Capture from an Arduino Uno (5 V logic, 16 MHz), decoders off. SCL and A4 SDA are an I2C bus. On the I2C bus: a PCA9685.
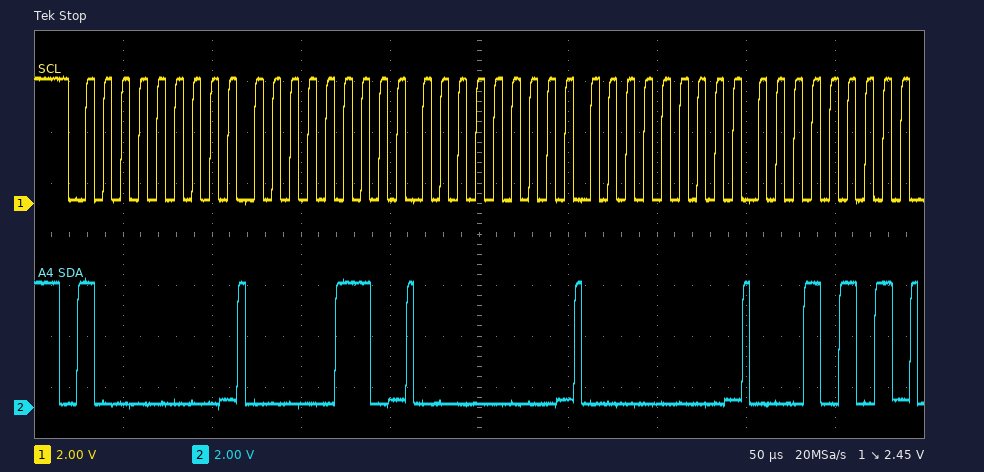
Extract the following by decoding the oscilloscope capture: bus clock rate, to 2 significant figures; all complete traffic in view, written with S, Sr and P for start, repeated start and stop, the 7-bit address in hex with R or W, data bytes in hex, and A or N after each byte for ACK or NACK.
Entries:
100 kHz
S 40W A 06 A 00 A 00 A 15 A
